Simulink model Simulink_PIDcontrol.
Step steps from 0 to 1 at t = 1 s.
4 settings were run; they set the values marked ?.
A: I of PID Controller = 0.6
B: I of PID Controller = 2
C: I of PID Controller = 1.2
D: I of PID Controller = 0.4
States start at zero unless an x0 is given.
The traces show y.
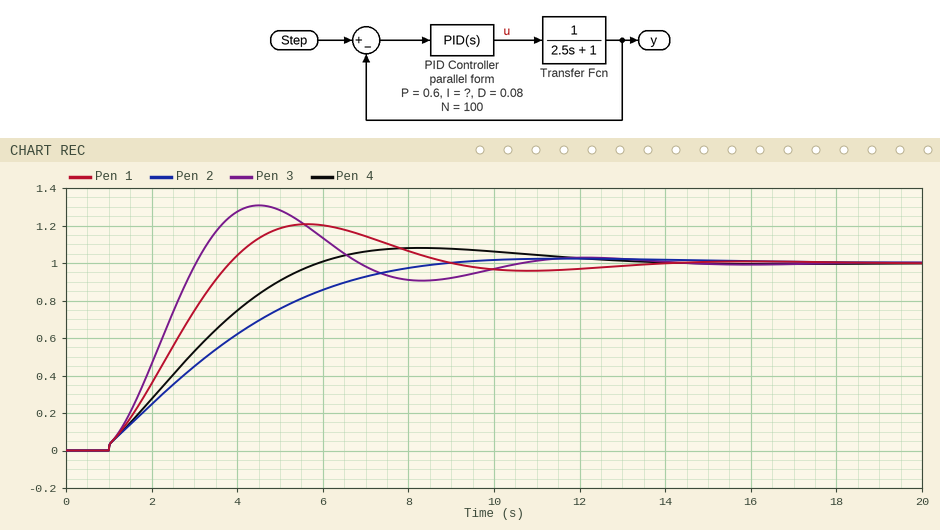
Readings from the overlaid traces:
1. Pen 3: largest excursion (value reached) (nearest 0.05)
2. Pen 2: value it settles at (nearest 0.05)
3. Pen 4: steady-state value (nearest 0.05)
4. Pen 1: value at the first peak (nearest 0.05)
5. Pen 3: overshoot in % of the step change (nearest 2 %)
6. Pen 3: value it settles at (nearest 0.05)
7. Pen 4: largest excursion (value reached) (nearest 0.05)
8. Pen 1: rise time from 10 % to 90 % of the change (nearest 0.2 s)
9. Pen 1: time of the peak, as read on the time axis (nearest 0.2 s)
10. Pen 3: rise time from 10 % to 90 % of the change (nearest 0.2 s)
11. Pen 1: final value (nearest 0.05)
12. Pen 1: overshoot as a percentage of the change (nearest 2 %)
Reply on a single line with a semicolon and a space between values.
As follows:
1.30; 1.00; 1.00; 1.20; 30 %; 1.00; 1.10; 2.2 s; 5.6 s; 1.6 s; 1.00; 20 %
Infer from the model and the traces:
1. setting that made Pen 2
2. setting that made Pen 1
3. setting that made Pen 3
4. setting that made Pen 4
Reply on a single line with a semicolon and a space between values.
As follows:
D; C; B; A
